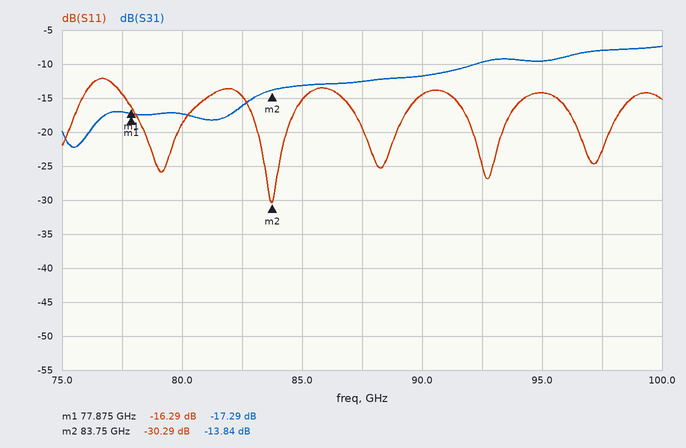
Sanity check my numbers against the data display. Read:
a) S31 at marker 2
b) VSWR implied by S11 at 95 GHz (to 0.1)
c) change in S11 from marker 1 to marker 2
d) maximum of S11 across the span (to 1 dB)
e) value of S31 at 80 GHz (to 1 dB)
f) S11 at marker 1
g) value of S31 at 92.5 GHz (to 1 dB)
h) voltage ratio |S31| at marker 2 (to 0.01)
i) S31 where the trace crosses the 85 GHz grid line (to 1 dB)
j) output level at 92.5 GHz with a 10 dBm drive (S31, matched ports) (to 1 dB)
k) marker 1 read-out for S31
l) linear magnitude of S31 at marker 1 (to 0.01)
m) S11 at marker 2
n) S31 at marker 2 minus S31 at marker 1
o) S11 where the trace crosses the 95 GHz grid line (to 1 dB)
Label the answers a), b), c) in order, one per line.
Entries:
a) -13.84 dB
b) 1.5
c) -14.00 dB
d) -12 dB
e) -17 dB
f) -16.29 dB
g) -10 dB
h) 0.20
i) -13 dB
j) 0 dBm
k) -17.29 dB
l) 0.14
m) -30.29 dB
n) 3.45 dB
o) -14 dB
